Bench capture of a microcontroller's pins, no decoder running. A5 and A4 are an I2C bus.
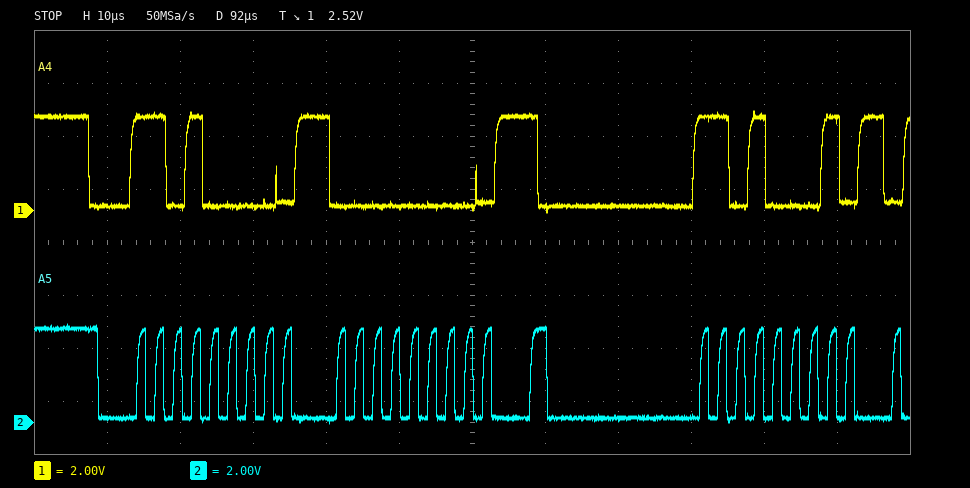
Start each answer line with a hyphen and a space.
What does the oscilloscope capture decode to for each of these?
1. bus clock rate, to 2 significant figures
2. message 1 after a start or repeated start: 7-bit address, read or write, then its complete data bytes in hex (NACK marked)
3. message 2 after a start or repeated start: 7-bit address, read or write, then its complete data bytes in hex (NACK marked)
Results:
- 400 kHz
- 0x68 write: 00
- 0x68 read
